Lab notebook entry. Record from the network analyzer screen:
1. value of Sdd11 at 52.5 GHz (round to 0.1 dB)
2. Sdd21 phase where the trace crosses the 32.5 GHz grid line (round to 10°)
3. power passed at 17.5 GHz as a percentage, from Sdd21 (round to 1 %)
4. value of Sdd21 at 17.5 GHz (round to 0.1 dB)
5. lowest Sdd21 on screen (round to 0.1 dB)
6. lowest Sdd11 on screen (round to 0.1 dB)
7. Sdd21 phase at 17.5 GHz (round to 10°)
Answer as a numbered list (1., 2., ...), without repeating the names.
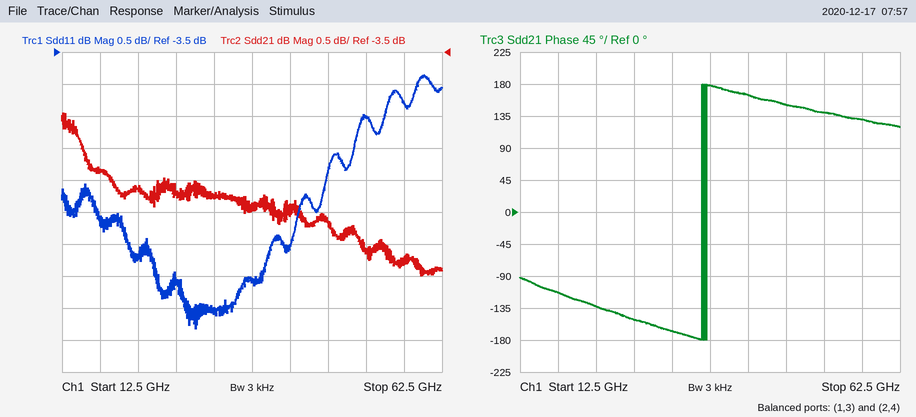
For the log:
1. -4.5 dB
2. -170°
3. 29 %
4. -5.4 dB
5. -7.0 dB
6. -7.8 dB
7. -110°
